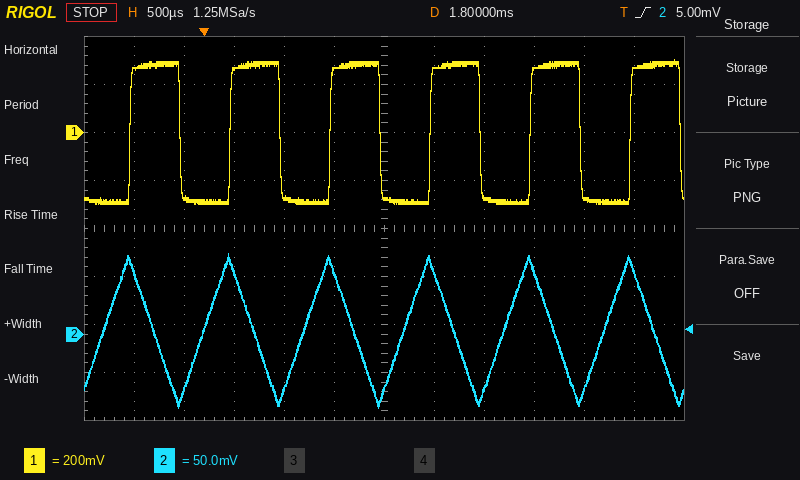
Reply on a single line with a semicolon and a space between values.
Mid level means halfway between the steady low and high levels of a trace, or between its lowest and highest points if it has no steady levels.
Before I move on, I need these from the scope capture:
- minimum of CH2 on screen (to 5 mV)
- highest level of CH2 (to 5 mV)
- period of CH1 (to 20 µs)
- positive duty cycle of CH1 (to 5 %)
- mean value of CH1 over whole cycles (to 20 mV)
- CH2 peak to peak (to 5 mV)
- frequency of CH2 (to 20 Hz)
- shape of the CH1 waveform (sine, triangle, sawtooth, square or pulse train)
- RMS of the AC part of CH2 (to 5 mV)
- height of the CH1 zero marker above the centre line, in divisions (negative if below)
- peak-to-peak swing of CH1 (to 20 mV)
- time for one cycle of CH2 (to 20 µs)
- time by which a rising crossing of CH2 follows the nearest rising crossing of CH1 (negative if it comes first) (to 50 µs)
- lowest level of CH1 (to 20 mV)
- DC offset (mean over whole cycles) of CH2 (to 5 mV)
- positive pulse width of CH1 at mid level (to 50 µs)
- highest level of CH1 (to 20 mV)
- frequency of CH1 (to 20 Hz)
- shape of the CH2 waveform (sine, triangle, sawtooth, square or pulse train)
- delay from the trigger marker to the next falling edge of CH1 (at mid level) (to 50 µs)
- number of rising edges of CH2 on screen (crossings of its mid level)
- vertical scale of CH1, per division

-75 mV; 85 mV; 1.00 ms; 50 %; 0 mV; 160 mV; 1.00 kHz; square; 45 mV; +2.0 div; 600 mV; 1.00 ms; -250 µs; -300 mV; 5 mV; 500 µs; 300 mV; 1.00 kHz; triangle; 750 µs; 6; 200 mV
